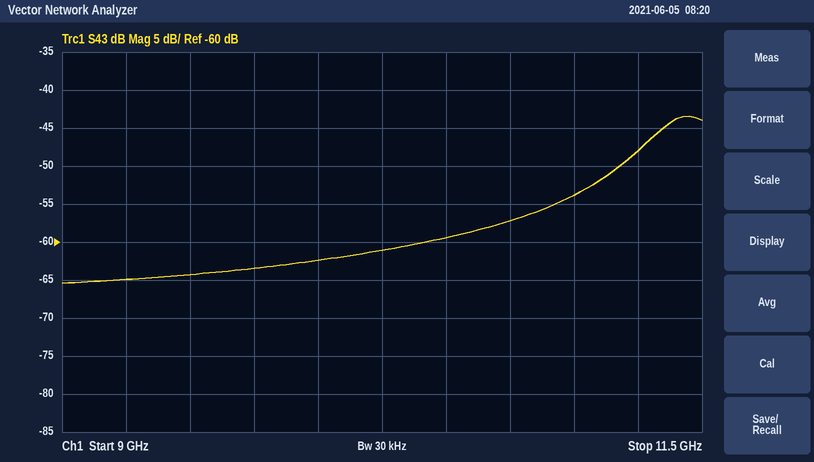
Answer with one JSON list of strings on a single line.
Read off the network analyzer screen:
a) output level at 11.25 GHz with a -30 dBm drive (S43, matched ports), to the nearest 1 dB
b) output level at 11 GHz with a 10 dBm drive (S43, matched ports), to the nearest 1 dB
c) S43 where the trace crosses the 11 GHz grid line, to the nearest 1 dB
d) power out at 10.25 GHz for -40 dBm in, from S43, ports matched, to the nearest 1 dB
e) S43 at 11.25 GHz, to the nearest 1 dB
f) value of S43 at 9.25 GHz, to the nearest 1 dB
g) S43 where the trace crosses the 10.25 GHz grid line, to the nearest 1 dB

["-78 dBm", "-44 dBm", "-54 dB", "-101 dBm", "-48 dB", "-65 dB", "-61 dB"]
